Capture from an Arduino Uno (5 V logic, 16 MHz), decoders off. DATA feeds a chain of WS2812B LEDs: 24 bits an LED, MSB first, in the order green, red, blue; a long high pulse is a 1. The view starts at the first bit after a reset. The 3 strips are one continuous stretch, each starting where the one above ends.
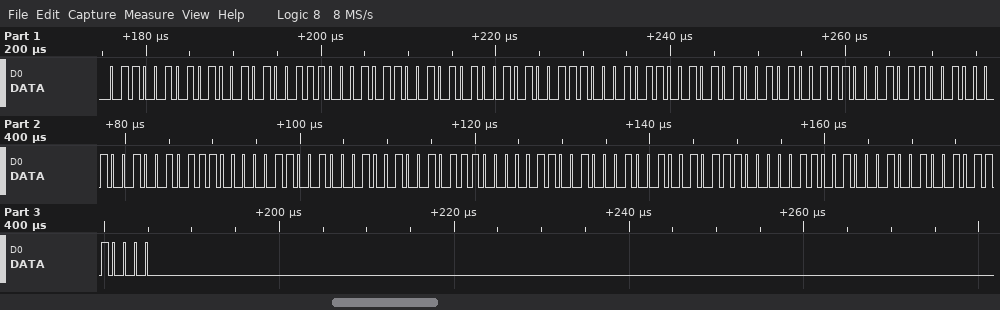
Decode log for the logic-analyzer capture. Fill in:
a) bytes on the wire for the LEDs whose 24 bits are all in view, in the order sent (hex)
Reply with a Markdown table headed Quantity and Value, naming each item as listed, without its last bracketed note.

| Quantity | Value |
|---|---|
| bytes on the wire for the LEDs whose 24 bits are all in view, in the order sent | 65 4A 71 65 4A 71 65 4A 71 64 49 70 64 49 70 64 49 70 64 49 70 |
